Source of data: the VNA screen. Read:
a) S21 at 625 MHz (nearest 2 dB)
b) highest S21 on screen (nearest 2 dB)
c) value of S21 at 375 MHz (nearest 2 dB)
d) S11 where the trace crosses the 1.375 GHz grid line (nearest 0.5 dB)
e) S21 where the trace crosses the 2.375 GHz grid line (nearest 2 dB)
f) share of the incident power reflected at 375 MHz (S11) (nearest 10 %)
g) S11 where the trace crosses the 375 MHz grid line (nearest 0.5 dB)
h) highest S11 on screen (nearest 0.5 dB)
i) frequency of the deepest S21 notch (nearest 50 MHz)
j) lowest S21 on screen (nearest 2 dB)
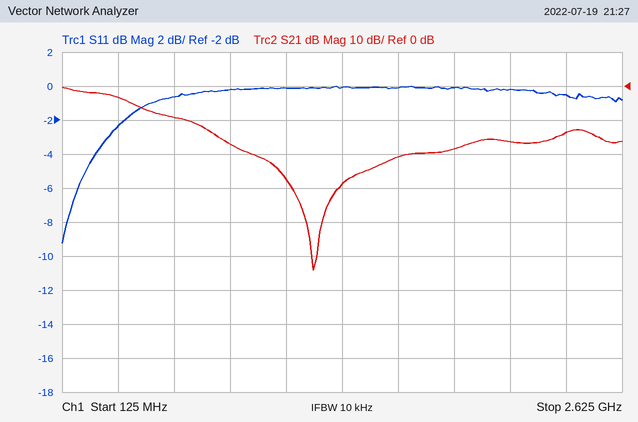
-10 dB
0 dB
-4 dB
0.0 dB
-14 dB
60 %
-2.5 dB
0.0 dB
1.25 GHz
-54 dB
